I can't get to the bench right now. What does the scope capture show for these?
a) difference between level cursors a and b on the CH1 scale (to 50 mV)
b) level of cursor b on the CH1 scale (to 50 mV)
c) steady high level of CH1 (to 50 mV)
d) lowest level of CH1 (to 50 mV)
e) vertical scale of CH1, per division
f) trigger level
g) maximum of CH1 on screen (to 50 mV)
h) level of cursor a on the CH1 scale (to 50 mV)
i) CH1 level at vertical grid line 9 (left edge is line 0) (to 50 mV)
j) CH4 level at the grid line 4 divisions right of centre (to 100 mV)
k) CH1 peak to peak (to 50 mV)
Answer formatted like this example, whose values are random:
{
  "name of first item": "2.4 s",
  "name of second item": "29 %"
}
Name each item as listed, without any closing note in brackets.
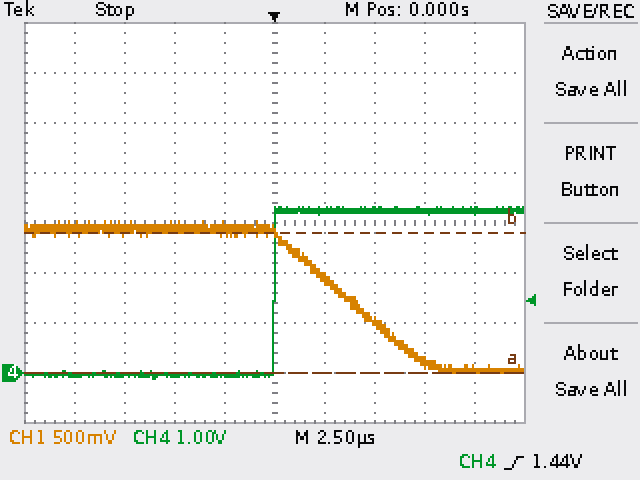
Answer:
{
  "difference between level cursors a and b on the CH1 scale": "1.40 V",
  "level of cursor b on the CH1 scale": "1.40 V",
  "steady high level of CH1": "1.45 V",
  "lowest level of CH1": "0 mV",
  "vertical scale of CH1, per division": "500 mV",
  "trigger level": "1.44 V",
  "maximum of CH1 on screen": "1.50 V",
  "level of cursor a on the CH1 scale": "0 mV",
  "CH1 level at vertical grid line 9 (left edge is line 0)": "50 mV",
  "CH4 level at the grid line 4 divisions right of centre": "3.2 V",
  "CH1 peak to peak": "1.50 V"
}
